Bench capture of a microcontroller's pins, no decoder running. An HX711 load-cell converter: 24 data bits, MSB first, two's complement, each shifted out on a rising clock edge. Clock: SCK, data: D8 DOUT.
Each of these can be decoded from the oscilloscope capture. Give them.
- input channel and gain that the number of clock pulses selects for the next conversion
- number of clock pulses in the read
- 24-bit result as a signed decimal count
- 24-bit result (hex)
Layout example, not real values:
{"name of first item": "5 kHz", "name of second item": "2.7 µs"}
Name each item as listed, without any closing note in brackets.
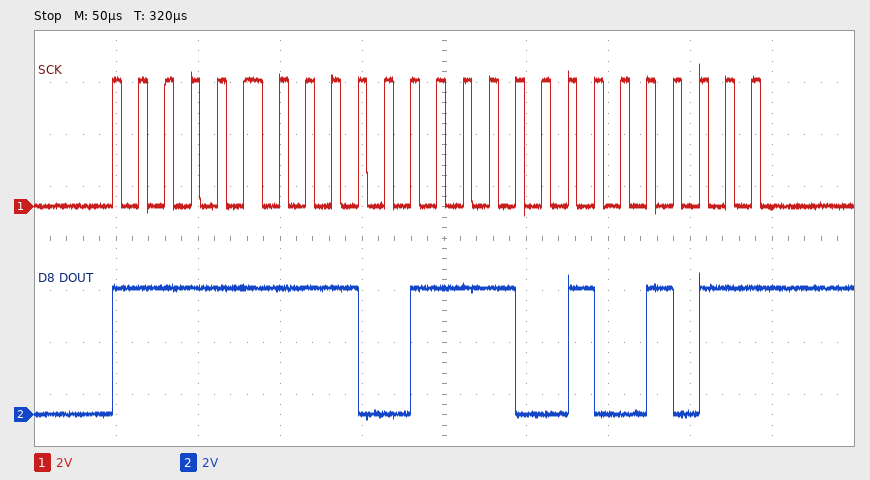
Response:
{"input channel and gain that the number of clock pulses selects for the next conversion": "channel A, gain 128", "number of clock pulses in the read": "25", "24-bit result as a signed decimal count": "-25013", "24-bit result": "0xFF9E4B"}
